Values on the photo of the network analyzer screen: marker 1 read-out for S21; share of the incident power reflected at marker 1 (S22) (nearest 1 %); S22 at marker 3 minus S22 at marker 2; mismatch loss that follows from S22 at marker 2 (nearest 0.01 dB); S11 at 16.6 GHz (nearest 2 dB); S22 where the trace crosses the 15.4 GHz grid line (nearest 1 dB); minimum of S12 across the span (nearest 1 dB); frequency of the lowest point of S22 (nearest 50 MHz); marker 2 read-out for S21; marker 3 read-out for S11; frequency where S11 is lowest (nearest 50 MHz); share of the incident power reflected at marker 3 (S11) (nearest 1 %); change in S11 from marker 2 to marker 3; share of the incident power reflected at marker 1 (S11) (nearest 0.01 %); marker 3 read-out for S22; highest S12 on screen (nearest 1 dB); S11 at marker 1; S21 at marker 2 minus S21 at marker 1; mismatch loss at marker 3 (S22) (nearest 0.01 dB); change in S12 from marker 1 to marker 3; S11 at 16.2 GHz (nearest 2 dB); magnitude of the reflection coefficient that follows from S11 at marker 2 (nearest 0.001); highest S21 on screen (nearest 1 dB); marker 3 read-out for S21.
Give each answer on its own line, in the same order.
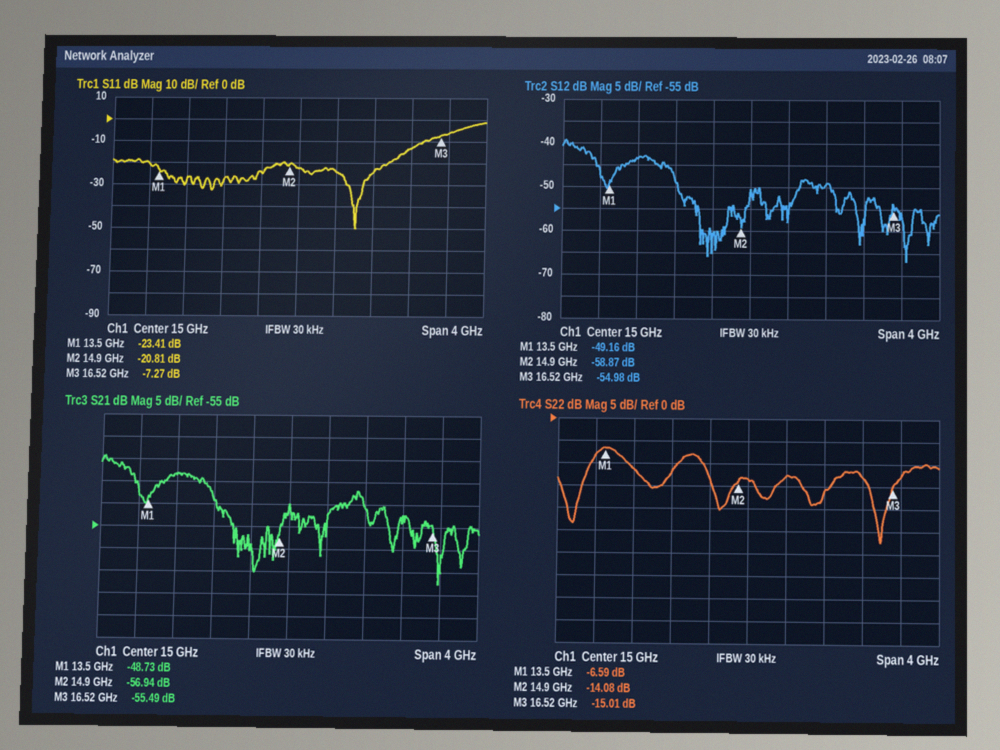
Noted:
-48.73 dB
22 %
-0.93 dB
0.17 dB
-6 dB
-13 dB
-67 dB
16.40 GHz
-56.94 dB
-7.27 dB
15.60 GHz
19 %
13.54 dB
0.46 %
-15.01 dB
-39 dB
-23.41 dB
-8.21 dB
0.14 dB
-5.82 dB
-14 dB
0.091
-39 dB
-55.49 dB
